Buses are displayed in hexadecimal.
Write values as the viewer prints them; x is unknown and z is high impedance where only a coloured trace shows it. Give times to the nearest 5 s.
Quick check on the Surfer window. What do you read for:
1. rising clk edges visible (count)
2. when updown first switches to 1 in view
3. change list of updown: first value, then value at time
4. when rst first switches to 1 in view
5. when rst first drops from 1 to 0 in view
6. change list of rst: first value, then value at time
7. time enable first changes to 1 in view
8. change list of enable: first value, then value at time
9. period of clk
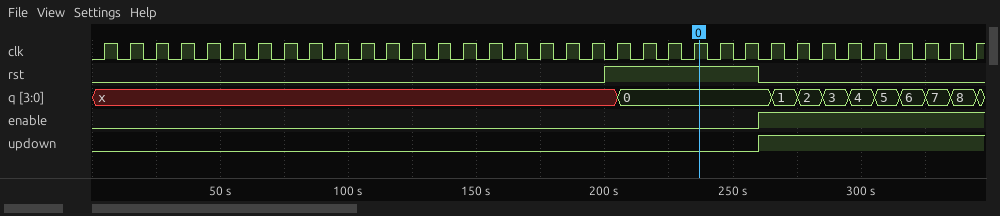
35
260 s
0, 1 at 260 s
200 s
260 s
0, 1 at 200 s, 0 at 260 s
260 s
0, 1 at 260 s
10 s
